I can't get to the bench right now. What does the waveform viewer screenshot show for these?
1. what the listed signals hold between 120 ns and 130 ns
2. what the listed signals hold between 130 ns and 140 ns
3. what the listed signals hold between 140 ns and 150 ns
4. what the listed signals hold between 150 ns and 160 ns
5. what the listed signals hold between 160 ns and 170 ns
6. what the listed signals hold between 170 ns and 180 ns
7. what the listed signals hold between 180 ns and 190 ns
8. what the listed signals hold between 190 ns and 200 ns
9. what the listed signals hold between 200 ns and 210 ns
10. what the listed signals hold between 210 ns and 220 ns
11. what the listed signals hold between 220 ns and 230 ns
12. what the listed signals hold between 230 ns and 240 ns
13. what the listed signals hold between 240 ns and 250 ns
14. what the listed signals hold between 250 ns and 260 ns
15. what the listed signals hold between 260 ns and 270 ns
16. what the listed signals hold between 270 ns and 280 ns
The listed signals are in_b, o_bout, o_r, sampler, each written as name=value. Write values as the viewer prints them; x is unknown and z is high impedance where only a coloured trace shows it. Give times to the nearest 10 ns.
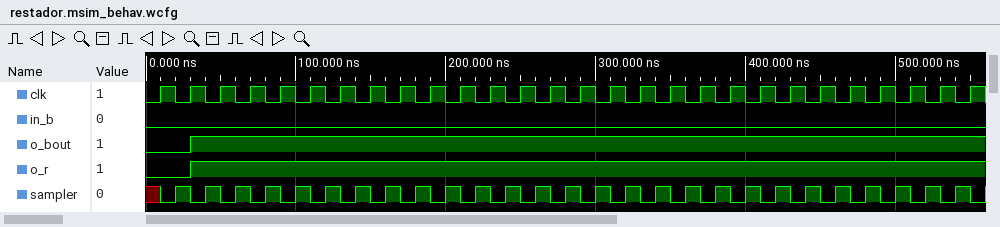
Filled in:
in_b=0, o_bout=1, o_r=1, sampler=1
in_b=0, o_bout=1, o_r=1, sampler=0
in_b=0, o_bout=1, o_r=1, sampler=1
in_b=0, o_bout=1, o_r=1, sampler=0
in_b=0, o_bout=1, o_r=1, sampler=1
in_b=0, o_bout=1, o_r=1, sampler=0
in_b=0, o_bout=1, o_r=1, sampler=1
in_b=0, o_bout=1, o_r=1, sampler=0
in_b=0, o_bout=1, o_r=1, sampler=1
in_b=0, o_bout=1, o_r=1, sampler=0
in_b=0, o_bout=1, o_r=1, sampler=1
in_b=0, o_bout=1, o_r=1, sampler=0
in_b=0, o_bout=1, o_r=1, sampler=1
in_b=0, o_bout=1, o_r=1, sampler=0
in_b=0, o_bout=1, o_r=1, sampler=1
in_b=0, o_bout=1, o_r=1, sampler=0
